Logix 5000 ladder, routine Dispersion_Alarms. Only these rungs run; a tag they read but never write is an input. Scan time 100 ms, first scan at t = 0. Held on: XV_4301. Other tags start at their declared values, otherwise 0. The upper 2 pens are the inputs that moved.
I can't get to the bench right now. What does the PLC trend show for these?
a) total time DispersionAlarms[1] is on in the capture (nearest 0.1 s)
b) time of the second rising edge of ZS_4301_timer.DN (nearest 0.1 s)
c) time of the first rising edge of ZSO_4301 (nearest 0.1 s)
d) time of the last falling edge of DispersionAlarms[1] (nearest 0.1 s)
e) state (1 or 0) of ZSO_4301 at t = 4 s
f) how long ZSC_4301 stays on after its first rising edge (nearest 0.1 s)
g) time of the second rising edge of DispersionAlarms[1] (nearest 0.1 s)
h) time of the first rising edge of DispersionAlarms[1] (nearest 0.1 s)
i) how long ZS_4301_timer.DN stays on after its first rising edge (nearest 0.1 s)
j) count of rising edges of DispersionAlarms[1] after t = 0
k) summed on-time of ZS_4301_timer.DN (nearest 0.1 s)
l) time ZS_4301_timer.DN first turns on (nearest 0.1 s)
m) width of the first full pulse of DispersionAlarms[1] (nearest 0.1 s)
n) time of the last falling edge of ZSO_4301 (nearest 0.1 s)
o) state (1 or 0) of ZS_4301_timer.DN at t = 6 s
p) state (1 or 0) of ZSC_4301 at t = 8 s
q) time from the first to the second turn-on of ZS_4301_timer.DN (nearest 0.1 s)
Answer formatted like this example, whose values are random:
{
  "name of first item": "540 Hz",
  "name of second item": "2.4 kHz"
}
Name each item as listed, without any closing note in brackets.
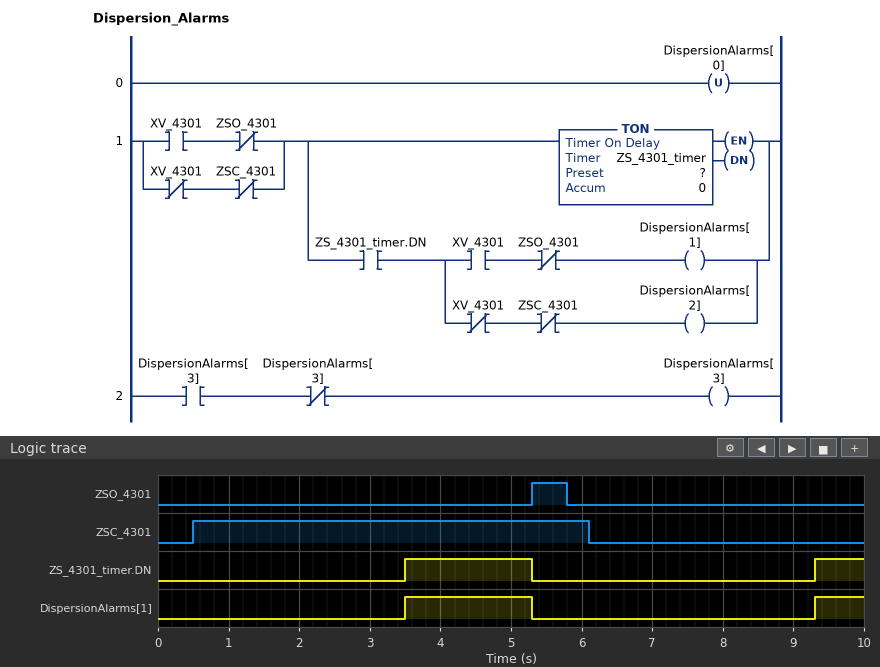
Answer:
{
  "total time DispersionAlarms[1] is on in the capture": "2.5 s",
  "time of the second rising edge of ZS_4301_timer.DN": "9.3 s",
  "time of the first rising edge of ZSO_4301": "5.3 s",
  "time of the last falling edge of DispersionAlarms[1]": "5.3 s",
  "state (1 or 0) of ZSO_4301 at t = 4 s": "0",
  "how long ZSC_4301 stays on after its first rising edge": "5.6 s",
  "time of the second rising edge of DispersionAlarms[1]": "9.3 s",
  "time of the first rising edge of DispersionAlarms[1]": "3.5 s",
  "how long ZS_4301_timer.DN stays on after its first rising edge": "1.8 s",
  "count of rising edges of DispersionAlarms[1] after t = 0": "2",
  "summed on-time of ZS_4301_timer.DN": "2.5 s",
  "time ZS_4301_timer.DN first turns on": "3.5 s",
  "width of the first full pulse of DispersionAlarms[1]": "1.8 s",
  "time of the last falling edge of ZSO_4301": "5.8 s",
  "state (1 or 0) of ZS_4301_timer.DN at t = 6 s": "0",
  "state (1 or 0) of ZSC_4301 at t = 8 s": "0",
  "time from the first to the second turn-on of ZS_4301_timer.DN": "5.8 s"
}
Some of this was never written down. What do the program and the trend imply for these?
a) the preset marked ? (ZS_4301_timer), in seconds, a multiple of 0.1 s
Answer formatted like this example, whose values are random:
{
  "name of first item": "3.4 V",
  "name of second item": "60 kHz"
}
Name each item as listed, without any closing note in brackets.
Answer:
{
  "the preset marked ? (ZS_4301_timer), in seconds, a multiple of 0.1 s": "3.5 s"
}
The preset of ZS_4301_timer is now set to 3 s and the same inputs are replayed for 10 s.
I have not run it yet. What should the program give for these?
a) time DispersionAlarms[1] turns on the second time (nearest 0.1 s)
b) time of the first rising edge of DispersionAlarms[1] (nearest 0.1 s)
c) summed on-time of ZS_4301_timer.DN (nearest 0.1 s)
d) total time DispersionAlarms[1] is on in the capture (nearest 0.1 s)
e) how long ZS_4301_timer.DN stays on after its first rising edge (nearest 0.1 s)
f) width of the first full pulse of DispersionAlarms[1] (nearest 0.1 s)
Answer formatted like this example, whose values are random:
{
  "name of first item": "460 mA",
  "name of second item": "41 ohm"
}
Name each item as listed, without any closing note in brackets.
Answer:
{
  "time DispersionAlarms[1] turns on the second time": "8.8 s",
  "time of the first rising edge of DispersionAlarms[1]": "3.0 s",
  "summed on-time of ZS_4301_timer.DN": "3.5 s",
  "total time DispersionAlarms[1] is on in the capture": "3.5 s",
  "how long ZS_4301_timer.DN stays on after its first rising edge": "2.3 s",
  "width of the first full pulse of DispersionAlarms[1]": "2.3 s"
}
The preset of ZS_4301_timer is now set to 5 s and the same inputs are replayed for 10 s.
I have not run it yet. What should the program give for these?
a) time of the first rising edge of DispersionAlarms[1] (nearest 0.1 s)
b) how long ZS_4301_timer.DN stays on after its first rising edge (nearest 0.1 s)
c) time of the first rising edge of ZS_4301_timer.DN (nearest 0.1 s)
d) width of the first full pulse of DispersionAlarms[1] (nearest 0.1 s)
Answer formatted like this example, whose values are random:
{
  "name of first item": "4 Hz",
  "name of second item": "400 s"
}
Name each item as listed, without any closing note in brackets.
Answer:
{
  "time of the first rising edge of DispersionAlarms[1]": "5.0 s",
  "how long ZS_4301_timer.DN stays on after its first rising edge": "0.3 s",
  "time of the first rising edge of ZS_4301_timer.DN": "5.0 s",
  "width of the first full pulse of DispersionAlarms[1]": "0.3 s"
}
